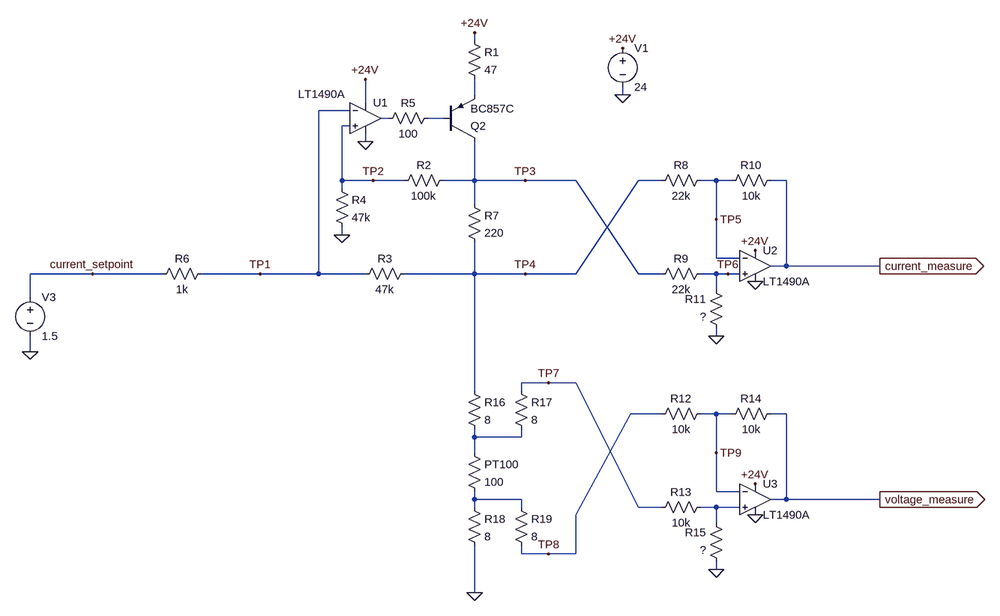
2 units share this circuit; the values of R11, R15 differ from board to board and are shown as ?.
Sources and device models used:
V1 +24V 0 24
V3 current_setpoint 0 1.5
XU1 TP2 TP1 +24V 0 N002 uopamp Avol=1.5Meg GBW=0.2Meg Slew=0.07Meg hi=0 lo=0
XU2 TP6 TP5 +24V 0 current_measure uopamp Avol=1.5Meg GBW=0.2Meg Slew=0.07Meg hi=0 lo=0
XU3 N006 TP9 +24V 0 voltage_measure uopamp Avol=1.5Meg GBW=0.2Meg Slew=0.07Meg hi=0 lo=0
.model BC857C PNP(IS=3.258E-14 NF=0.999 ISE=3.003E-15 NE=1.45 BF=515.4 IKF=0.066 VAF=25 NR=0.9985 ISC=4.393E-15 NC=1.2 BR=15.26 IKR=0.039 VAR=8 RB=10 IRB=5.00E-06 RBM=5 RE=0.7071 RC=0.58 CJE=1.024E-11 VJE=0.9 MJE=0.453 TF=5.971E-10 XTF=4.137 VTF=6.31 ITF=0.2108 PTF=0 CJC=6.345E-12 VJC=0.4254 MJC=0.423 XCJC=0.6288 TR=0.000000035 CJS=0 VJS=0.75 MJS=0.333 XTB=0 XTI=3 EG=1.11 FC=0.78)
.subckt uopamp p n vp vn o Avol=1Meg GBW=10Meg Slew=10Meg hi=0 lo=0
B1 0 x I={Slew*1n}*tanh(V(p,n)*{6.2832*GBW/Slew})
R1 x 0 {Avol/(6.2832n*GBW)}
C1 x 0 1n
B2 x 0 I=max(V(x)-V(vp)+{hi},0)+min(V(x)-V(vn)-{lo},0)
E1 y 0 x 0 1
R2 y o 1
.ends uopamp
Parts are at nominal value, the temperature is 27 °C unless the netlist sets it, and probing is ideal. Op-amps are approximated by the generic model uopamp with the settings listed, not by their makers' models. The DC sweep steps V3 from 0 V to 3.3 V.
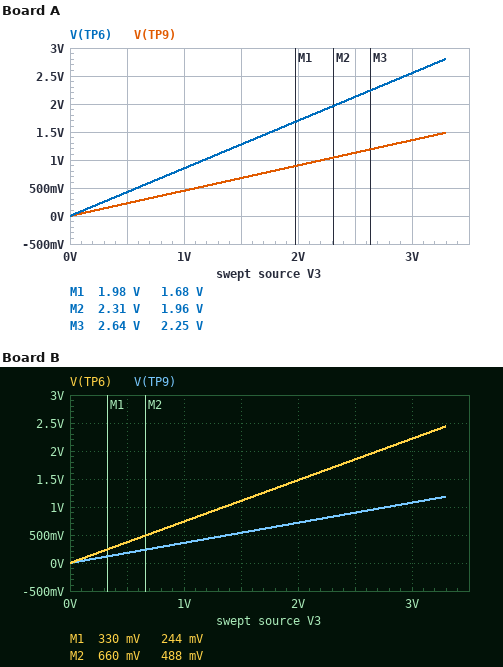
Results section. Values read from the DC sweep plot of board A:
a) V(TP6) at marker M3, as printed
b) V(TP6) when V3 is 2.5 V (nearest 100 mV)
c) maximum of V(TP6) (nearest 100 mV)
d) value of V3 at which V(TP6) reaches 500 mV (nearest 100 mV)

2.25 V
2.1 V
2.8 V
600 mV
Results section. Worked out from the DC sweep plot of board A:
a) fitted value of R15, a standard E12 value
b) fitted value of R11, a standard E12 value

8.2 kΩ
8.2 kΩ
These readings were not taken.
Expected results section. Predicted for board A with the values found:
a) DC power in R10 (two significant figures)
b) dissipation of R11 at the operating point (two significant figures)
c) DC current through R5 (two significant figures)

2.4 µW
200 µW
19 µA
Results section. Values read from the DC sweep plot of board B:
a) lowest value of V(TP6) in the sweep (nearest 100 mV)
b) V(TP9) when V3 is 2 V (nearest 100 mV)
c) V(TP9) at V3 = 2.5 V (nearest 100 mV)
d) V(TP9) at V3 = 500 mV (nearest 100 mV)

0 V
700 mV
900 mV
200 mV
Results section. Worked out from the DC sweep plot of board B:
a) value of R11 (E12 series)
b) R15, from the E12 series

6.8 kΩ
5.6 kΩ
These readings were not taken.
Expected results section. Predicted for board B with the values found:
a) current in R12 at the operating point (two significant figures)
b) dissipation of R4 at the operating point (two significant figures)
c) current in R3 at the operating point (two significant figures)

43 µA
48 µW
2.4 µA
